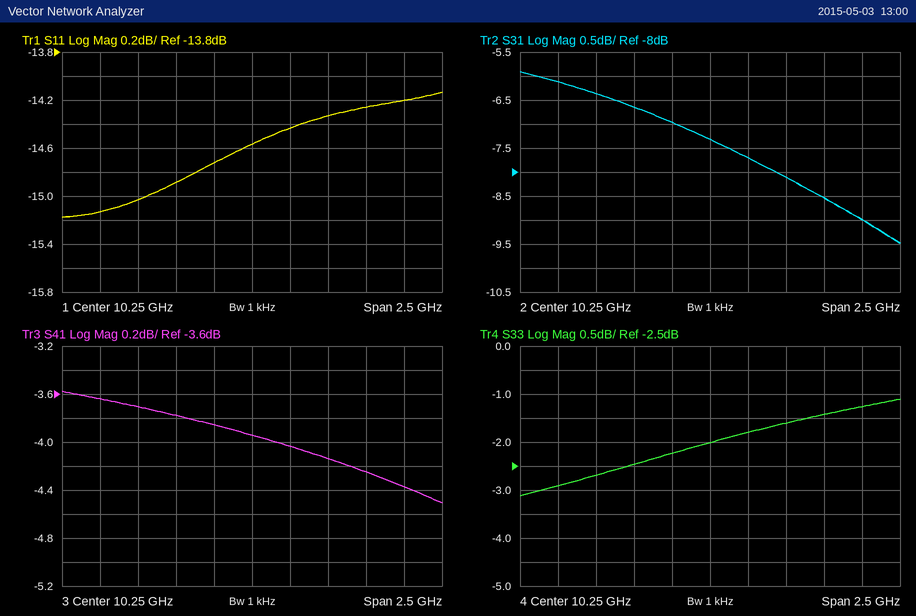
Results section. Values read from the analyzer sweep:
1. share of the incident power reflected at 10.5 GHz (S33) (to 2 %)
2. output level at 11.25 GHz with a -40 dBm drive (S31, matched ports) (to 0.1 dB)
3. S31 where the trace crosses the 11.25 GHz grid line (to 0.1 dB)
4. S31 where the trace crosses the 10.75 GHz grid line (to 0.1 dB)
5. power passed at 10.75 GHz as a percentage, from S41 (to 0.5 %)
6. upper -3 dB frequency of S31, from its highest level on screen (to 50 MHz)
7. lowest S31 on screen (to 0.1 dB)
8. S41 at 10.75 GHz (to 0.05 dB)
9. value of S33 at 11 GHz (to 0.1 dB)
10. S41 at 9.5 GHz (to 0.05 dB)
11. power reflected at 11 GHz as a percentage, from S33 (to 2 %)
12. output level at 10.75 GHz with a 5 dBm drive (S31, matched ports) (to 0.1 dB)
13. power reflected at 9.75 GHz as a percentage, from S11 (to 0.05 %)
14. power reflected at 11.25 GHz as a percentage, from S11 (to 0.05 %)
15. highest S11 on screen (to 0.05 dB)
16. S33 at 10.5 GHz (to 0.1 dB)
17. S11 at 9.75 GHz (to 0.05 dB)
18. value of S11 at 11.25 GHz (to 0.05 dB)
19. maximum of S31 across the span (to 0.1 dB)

66 %
-49.0 dBm
-9.0 dB
-8.1 dB
38.5 %
11.20 GHz
-9.5 dB
-4.15 dB
-1.4 dB
-3.70 dB
72 %
-3.1 dBm
3.25 %
3.80 %
-14.15 dB
-1.8 dB
-14.90 dB
-14.20 dB
-5.9 dB
